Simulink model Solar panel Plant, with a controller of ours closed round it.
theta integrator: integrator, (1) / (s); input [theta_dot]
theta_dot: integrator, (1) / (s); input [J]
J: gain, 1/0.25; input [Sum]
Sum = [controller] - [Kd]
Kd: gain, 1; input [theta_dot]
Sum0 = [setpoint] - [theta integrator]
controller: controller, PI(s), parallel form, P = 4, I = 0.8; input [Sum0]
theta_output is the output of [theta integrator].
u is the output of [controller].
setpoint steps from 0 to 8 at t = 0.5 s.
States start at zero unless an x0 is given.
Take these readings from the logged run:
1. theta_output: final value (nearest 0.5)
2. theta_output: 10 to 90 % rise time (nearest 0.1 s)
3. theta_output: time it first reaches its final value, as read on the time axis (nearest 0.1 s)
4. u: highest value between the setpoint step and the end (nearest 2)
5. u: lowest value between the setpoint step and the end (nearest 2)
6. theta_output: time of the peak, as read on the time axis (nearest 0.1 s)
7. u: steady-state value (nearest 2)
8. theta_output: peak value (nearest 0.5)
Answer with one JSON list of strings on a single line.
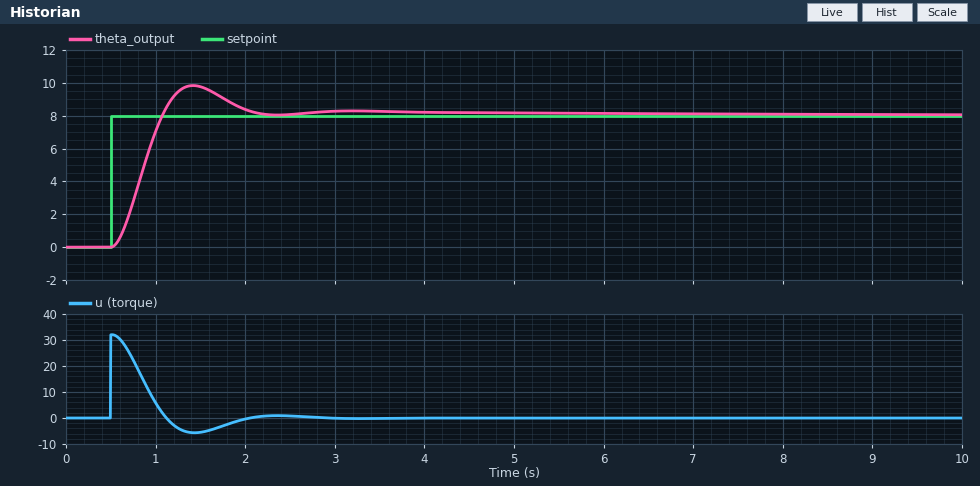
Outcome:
["8.0", "0.4 s", "1.1 s", "32", "-6", "1.4 s", "0", "10.0"]
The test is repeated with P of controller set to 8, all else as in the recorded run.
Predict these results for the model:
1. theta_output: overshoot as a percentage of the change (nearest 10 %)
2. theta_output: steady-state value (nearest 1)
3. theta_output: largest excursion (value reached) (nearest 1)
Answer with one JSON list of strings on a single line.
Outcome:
["30 %", "8", "11"]
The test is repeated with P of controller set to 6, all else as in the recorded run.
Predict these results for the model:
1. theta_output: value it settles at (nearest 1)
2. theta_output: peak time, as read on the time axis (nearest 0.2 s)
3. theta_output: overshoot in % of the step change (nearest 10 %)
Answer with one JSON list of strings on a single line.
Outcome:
["8", "1.2 s", "30 %"]
